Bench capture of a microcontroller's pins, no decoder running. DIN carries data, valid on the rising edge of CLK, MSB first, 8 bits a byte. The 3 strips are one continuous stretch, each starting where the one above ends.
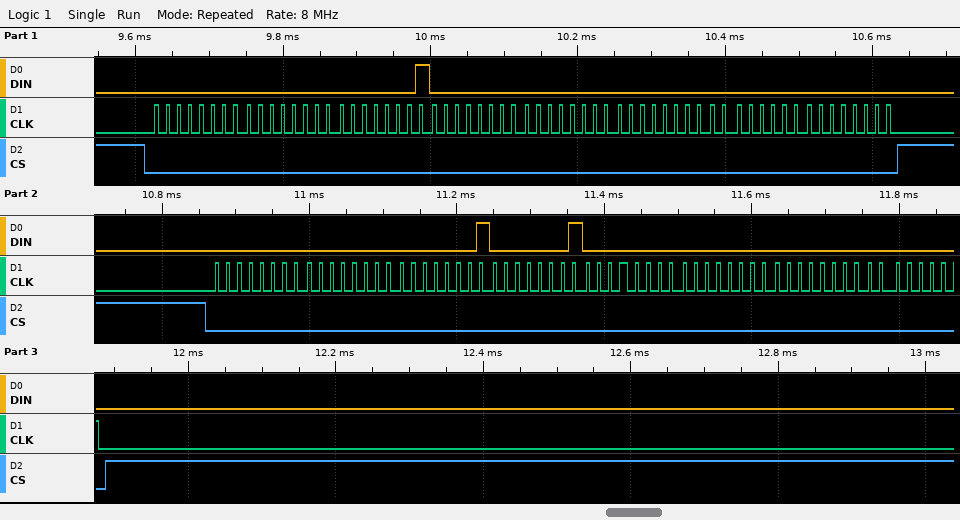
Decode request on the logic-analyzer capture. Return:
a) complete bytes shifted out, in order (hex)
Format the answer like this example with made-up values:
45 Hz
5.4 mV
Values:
0x00 0x00 0x01 0x00 0x00 0x00 0x00 0x00 0x00 0x00 0x01 0x01 0x00 0x00 0x00 0x00
